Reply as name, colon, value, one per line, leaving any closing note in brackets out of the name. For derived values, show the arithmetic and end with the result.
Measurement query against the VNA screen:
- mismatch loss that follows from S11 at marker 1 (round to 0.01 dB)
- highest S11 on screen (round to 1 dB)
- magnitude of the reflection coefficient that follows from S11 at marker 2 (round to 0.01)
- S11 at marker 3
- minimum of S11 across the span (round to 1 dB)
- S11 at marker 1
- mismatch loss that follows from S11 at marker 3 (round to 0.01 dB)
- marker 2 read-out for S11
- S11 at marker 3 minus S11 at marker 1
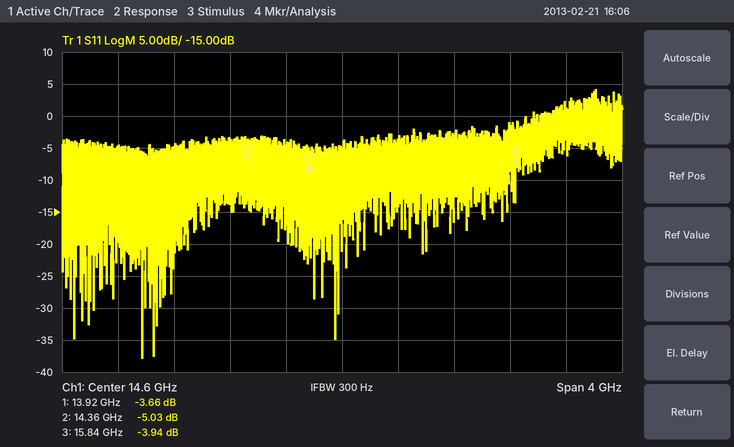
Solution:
mismatch loss that follows from S11 at marker 1: −10 log10(1 − 10^(-3.66/10)) ≈ 2.45 dB
highest S11 on screen: 4 dB
magnitude of the reflection coefficient that follows from S11 at marker 2: 10^(-5.03/20) ≈ 0.56
S11 at marker 3: -3.94 dB
minimum of S11 across the span: -38 dB
S11 at marker 1: -3.66 dB
mismatch loss that follows from S11 at marker 3: −10 log10(1 − 10^(-3.94/10)) ≈ 2.24 dB
marker 2 read-out for S11: -5.03 dB
S11 at marker 3 minus S11 at marker 1: -3.94 − (-3.66) = -0.28 dB
